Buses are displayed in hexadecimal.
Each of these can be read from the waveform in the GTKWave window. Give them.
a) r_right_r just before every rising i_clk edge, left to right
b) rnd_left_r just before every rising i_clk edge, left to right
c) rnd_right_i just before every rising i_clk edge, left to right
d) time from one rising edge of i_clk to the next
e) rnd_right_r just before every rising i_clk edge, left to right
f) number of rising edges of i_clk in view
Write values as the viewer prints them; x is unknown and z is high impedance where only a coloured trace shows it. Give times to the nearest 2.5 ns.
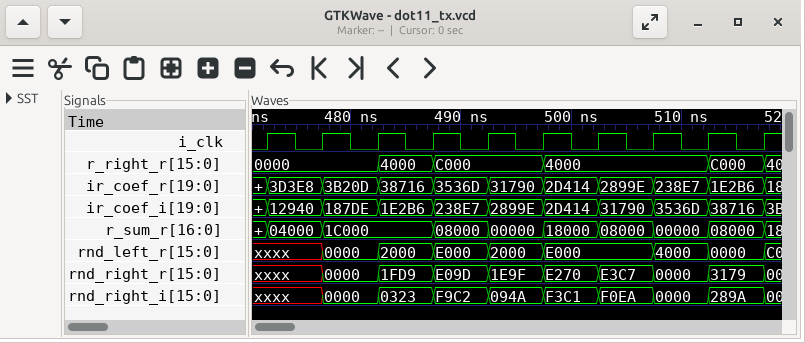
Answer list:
0000, 0000, 0000, 4000, C000, C000, 4000, 4000, 4000, C000
xxxx, xxxx, 0000, 2000, E000, 2000, E000, E000, 4000, 0000
xxxx, xxxx, 0000, 0323, F9C2, 094A, F3C1, F0EA, 0000, 289A
5 ns
xxxx, xxxx, 0000, 1FD9, E09D, 1E9F, E270, E3C7, 0000, 3179
10
